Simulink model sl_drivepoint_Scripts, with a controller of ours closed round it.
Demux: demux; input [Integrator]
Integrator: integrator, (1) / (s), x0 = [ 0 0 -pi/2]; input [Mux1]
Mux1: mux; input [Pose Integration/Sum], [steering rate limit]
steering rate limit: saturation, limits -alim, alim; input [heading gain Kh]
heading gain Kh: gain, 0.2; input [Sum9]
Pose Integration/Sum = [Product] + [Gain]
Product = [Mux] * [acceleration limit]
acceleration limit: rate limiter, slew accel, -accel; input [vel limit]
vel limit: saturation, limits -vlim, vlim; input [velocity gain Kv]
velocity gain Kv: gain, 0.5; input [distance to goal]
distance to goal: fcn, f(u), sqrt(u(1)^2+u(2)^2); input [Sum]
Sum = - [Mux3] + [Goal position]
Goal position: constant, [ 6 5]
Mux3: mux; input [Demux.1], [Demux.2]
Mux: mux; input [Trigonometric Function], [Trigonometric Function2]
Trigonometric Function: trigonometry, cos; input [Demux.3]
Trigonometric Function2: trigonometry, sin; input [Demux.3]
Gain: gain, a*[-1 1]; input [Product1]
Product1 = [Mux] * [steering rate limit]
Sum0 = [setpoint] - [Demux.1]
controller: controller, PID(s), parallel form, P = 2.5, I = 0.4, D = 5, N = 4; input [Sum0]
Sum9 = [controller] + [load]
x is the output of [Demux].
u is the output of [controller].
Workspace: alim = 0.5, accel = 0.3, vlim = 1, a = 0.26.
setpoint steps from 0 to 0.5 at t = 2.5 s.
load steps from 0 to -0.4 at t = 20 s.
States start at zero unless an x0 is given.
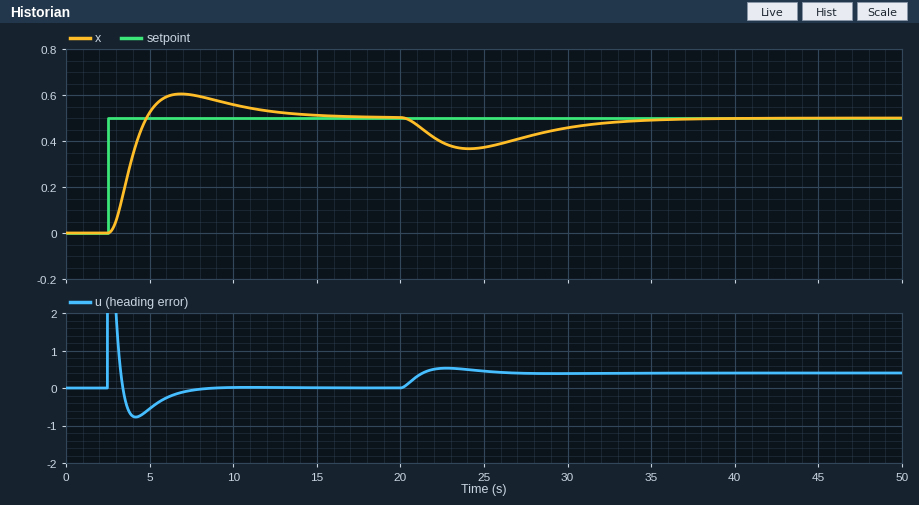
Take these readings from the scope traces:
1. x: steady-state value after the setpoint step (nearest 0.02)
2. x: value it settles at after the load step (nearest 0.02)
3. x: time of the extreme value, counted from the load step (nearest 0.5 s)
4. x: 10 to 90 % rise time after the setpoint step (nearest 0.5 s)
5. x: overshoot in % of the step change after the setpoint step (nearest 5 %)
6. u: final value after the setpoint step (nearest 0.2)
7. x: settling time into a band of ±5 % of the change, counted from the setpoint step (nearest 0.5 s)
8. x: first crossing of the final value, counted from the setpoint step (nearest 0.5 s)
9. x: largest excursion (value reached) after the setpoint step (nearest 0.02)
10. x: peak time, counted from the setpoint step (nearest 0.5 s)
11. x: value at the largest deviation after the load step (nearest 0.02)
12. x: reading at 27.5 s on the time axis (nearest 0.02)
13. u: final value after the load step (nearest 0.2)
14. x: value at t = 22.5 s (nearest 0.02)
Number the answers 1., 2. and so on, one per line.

1. 0.50
2. 0.50
3. 4.0 s
4. 1.5 s
5. 20 %
6. 0.0
7. 10.0 s
8. 2.5 s
9. 0.60
10. 4.5 s
11. 0.36
12. 0.42
13. 0.4
14. 0.40
